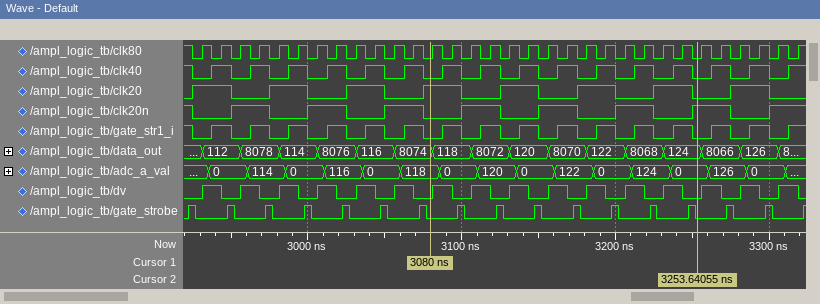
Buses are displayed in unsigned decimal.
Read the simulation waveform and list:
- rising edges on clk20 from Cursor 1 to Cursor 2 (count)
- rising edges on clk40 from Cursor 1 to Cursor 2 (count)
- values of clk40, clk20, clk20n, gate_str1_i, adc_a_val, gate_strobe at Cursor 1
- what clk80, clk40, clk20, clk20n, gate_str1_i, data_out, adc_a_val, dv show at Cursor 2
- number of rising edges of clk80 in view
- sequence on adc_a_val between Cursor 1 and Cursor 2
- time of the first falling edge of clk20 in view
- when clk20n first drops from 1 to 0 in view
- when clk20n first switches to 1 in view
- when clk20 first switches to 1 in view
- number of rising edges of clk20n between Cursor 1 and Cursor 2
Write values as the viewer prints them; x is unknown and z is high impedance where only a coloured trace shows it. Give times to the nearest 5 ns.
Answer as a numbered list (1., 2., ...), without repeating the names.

1. 3
2. 7
3. clk40=0, clk20=1, clk20n=0, gate_str1_i=0, adc_a_val=118, gate_strobe=0
4. clk80=0, clk40=0, clk20=0, clk20n=1, gate_str1_i=0, data_out=124, adc_a_val=0, dv=0
5. 32
6. 118, 0, 120, 0, 122, 0, 124, 0
7. 2950 ns
8. 2925 ns
9. 2950 ns
10. 2925 ns
11. 4
